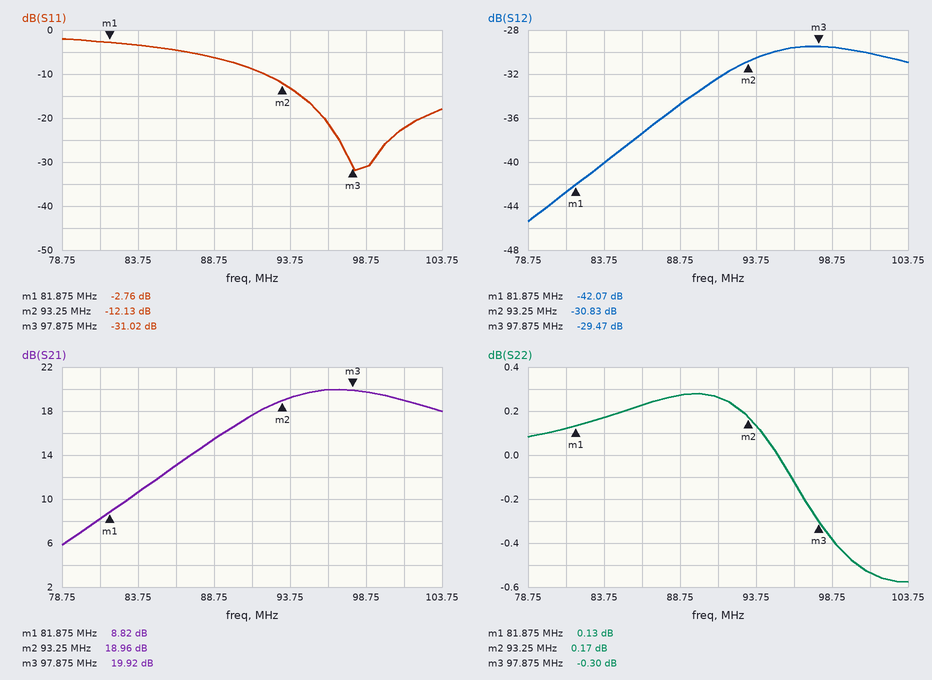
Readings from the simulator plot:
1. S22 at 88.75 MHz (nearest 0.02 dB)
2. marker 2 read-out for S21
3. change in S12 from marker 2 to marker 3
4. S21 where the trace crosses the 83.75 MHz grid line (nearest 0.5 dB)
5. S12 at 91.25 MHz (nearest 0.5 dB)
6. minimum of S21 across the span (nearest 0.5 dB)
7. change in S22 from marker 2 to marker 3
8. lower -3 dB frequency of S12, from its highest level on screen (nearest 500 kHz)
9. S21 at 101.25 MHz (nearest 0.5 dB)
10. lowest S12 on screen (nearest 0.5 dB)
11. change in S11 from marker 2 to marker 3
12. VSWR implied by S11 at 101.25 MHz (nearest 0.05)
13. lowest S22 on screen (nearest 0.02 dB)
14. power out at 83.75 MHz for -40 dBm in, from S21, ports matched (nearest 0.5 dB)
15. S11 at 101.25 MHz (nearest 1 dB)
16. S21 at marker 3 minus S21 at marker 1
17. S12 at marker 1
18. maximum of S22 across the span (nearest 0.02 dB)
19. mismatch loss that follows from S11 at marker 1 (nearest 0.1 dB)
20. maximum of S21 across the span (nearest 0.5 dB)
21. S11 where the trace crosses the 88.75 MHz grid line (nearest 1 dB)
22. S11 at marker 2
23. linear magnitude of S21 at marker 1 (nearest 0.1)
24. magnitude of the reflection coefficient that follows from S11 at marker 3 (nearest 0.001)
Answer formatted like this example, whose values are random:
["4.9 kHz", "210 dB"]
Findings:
["0.28 dB", "18.96 dB", "1.36 dB", "10.5 dB", "-32.5 dB", "6.0 dB", "-0.47 dB", "91.0 MHz", "19.0 dB", "-45.5 dB", "-18.89 dB", "1.15", "-0.58 dB", "-29.5 dBm", "-22 dB", "11.10 dB", "-42.07 dB", "0.28 dB", "3.3 dB", "20.0 dB", "-6 dB", "-12.13 dB", "2.8", "0.028"]
